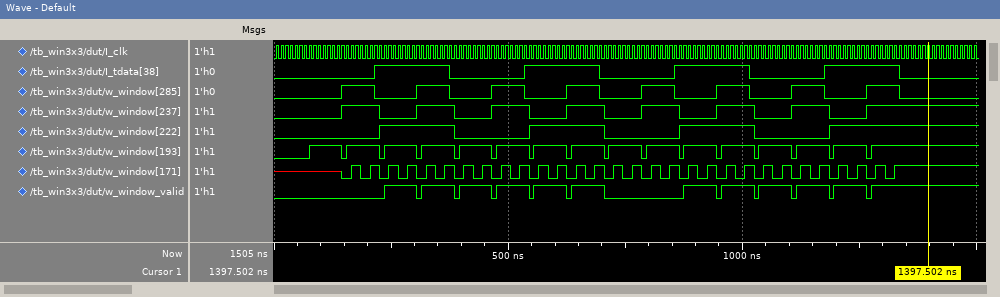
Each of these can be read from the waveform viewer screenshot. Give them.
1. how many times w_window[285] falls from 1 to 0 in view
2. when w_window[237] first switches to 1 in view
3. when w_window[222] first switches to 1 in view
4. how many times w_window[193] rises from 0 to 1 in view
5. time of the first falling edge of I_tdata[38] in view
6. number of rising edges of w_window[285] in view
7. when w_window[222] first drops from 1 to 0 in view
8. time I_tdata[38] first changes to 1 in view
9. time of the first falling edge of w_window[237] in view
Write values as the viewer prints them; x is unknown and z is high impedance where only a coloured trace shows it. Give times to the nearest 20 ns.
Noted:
8
140 ns
220 ns
16
380 ns
8
380 ns
220 ns
220 ns
